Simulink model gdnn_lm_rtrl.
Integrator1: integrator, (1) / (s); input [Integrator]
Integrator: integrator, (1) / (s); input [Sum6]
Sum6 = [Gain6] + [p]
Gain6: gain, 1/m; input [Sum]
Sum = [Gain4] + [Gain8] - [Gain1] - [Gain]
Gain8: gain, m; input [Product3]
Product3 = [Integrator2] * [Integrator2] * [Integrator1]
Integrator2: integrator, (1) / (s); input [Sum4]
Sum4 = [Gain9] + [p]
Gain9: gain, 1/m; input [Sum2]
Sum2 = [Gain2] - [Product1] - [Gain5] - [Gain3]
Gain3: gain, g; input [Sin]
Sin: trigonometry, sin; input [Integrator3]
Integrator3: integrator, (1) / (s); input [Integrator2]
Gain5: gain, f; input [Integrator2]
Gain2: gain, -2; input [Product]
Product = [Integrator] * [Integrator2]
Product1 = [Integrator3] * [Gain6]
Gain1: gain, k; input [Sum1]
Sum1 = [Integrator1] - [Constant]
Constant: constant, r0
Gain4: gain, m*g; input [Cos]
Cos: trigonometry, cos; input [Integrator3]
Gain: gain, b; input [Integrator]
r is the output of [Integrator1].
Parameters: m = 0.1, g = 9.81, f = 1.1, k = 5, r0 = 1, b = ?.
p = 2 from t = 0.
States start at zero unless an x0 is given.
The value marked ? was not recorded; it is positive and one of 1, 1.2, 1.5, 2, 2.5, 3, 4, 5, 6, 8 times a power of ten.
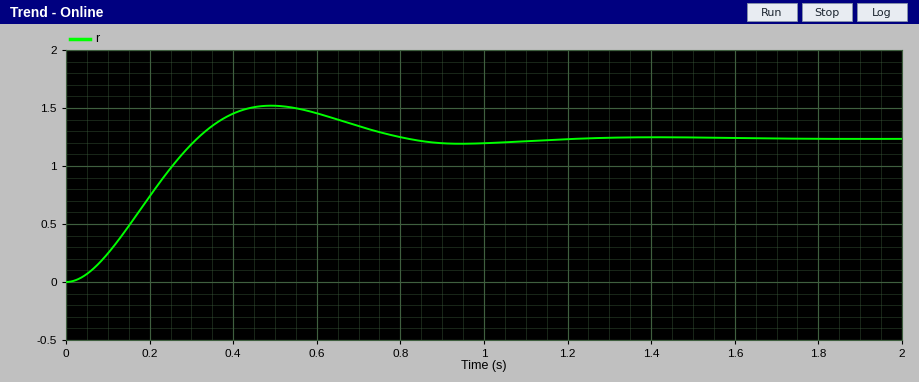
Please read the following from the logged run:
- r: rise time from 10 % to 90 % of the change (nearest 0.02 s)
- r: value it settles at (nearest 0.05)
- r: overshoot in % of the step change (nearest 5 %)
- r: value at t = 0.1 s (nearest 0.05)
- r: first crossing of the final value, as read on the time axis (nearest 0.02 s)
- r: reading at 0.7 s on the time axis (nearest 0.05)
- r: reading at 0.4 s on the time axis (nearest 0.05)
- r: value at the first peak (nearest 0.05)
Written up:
0.22 s
1.25
25 %
0.25
0.32 s
1.35
1.45
1.50
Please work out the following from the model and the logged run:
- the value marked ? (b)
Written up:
0.6
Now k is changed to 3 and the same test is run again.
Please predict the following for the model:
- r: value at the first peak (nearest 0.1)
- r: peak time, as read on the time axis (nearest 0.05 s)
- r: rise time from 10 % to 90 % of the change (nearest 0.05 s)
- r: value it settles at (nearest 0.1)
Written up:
1.6
0.70 s
0.30 s
1.4
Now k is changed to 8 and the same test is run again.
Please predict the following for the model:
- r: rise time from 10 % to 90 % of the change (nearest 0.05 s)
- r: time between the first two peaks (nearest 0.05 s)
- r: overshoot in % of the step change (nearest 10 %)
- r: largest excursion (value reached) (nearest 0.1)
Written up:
0.15 s
0.55 s
30 %
1.5
